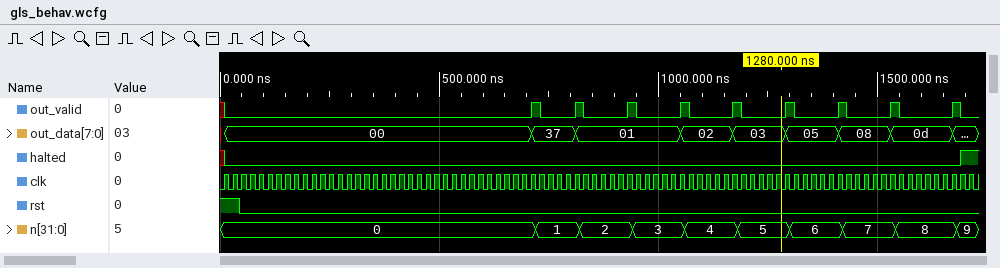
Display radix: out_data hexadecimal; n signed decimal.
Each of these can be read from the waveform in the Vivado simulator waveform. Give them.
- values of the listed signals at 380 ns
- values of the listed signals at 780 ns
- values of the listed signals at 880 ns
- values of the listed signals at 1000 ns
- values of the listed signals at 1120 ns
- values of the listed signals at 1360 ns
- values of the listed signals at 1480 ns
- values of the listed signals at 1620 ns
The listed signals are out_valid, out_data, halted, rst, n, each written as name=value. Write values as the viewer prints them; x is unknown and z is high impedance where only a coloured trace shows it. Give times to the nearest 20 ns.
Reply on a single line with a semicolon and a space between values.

out_valid=0, out_data=00, halted=0, rst=0, n=0; out_valid=0, out_data=37, halted=0, rst=0, n=1; out_valid=0, out_data=01, halted=0, rst=0, n=2; out_valid=0, out_data=01, halted=0, rst=0, n=3; out_valid=0, out_data=02, halted=0, rst=0, n=4; out_valid=0, out_data=05, halted=0, rst=0, n=6; out_valid=0, out_data=08, halted=0, rst=0, n=7; out_valid=0, out_data=0d, halted=0, rst=0, n=8
